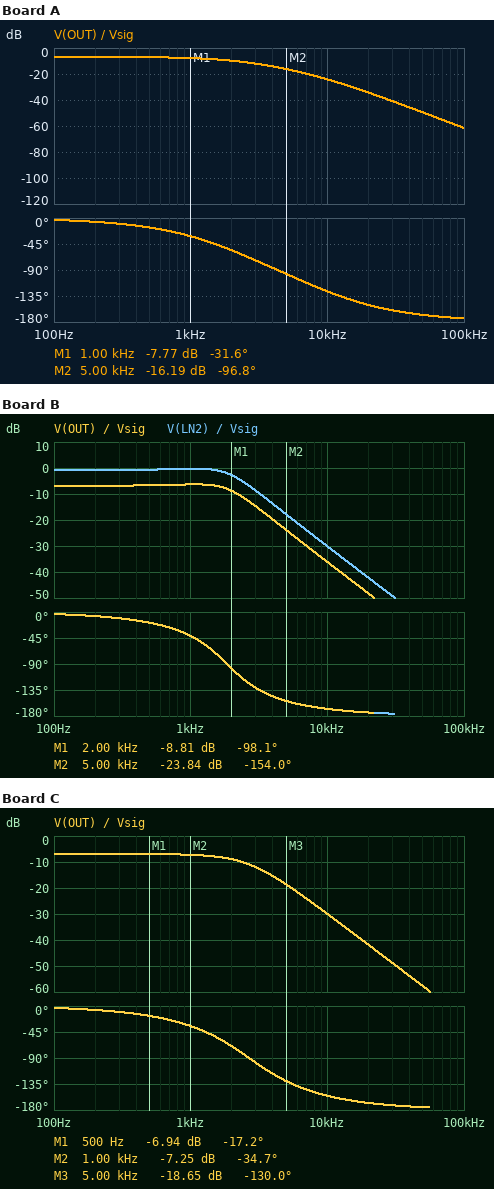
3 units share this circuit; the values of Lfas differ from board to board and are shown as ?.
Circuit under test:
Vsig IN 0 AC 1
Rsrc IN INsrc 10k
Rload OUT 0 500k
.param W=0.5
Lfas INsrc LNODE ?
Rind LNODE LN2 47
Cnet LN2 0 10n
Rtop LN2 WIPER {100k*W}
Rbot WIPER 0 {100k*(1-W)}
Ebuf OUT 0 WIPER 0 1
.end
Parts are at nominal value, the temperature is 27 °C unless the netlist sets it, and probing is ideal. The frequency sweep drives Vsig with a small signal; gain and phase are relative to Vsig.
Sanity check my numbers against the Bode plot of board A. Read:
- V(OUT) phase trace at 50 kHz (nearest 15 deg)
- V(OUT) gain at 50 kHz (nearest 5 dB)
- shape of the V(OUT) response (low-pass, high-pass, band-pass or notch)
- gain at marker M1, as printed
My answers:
-165 deg
-50 dB
low-pass
-7.77 dB
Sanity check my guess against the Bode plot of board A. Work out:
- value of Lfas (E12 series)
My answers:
150 mH
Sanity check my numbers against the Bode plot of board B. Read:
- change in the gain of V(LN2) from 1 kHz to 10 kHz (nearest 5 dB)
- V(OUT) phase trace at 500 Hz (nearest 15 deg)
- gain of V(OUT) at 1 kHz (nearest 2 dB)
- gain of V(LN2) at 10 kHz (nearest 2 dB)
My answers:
-30 dB
-15 deg
-6 dB
-30 dB
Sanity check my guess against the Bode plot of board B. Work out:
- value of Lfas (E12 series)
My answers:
820 mH
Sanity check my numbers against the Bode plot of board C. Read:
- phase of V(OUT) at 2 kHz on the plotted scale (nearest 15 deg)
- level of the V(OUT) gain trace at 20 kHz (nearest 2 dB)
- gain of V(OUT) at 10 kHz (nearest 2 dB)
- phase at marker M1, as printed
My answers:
-75 deg
-42 dB
-30 dB
-17.2 deg
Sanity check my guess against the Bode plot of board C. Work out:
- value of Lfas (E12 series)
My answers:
390 mH
